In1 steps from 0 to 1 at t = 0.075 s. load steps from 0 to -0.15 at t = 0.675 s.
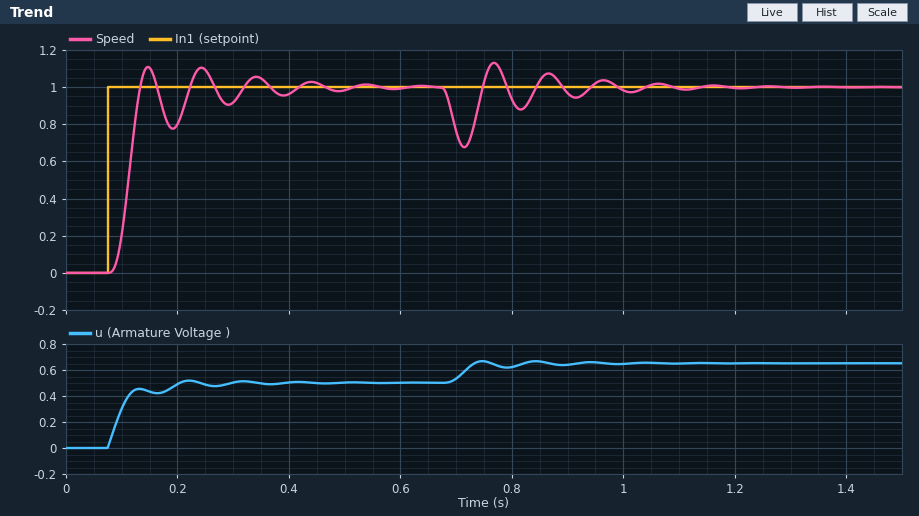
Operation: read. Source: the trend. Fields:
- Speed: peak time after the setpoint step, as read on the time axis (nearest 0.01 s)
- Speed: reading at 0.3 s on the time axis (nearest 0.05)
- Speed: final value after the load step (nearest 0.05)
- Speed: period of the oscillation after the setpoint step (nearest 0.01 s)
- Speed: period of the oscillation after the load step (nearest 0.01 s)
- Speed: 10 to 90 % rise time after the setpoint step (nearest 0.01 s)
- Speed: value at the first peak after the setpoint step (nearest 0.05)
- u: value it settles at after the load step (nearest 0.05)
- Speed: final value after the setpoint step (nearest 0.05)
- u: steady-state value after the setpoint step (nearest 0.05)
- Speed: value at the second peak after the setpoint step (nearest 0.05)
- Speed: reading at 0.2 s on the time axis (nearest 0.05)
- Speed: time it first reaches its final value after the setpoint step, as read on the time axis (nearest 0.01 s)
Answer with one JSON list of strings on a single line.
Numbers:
["0.15 s", "0.90", "1.00", "0.10 s", "0.10 s", "0.03 s", "1.10", "0.65", "1.00", "0.50", "1.10", "0.80", "0.13 s"]
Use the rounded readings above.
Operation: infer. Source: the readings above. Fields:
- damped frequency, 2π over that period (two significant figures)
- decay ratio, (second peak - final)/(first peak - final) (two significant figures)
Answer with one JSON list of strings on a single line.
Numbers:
["63 rad/s", "1.0"]
